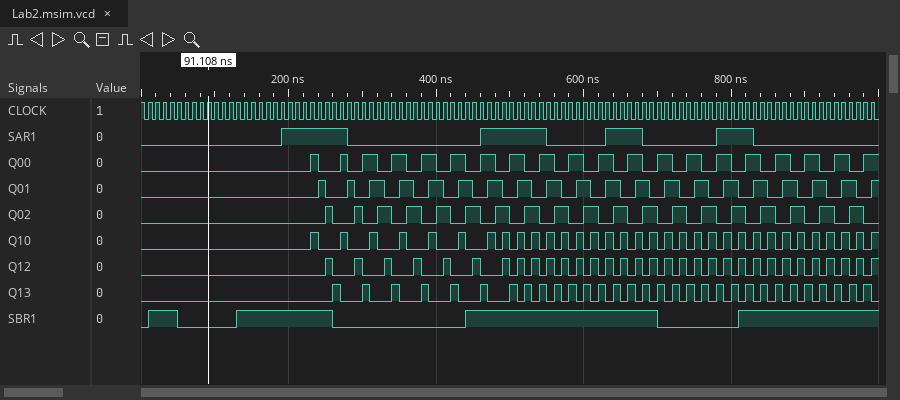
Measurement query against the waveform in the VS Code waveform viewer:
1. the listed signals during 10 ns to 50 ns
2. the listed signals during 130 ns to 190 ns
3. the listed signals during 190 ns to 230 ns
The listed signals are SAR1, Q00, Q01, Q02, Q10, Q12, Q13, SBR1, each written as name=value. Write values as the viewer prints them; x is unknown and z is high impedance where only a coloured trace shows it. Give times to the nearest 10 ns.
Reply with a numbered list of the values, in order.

1. SAR1=0, Q00=0, Q01=0, Q02=0, Q10=0, Q12=0, Q13=0, SBR1=1
2. SAR1=0, Q00=0, Q01=0, Q02=0, Q10=0, Q12=0, Q13=0, SBR1=1
3. SAR1=1, Q00=0, Q01=0, Q02=0, Q10=0, Q12=0, Q13=0, SBR1=1
